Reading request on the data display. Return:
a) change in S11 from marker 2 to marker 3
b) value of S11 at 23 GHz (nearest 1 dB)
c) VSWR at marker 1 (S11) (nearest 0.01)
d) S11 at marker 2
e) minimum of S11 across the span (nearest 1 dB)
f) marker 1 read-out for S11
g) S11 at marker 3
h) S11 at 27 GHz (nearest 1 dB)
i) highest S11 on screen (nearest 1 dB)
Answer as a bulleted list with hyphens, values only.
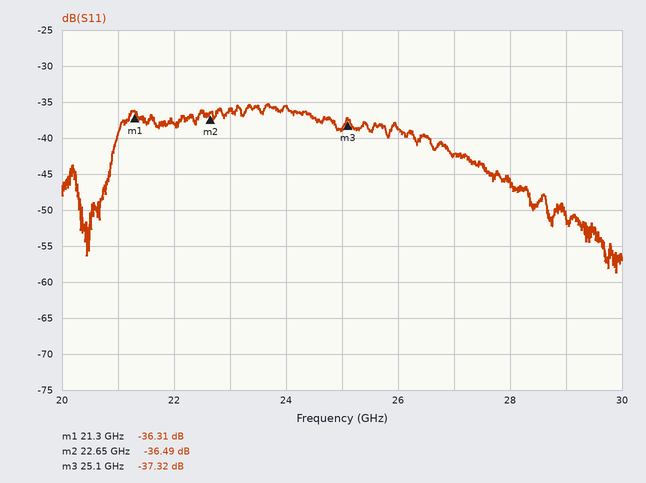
- -0.83 dB
- -36 dB
- 1.03
- -36.49 dB
- -59 dB
- -36.31 dB
- -37.32 dB
- -42 dB
- -35 dB
